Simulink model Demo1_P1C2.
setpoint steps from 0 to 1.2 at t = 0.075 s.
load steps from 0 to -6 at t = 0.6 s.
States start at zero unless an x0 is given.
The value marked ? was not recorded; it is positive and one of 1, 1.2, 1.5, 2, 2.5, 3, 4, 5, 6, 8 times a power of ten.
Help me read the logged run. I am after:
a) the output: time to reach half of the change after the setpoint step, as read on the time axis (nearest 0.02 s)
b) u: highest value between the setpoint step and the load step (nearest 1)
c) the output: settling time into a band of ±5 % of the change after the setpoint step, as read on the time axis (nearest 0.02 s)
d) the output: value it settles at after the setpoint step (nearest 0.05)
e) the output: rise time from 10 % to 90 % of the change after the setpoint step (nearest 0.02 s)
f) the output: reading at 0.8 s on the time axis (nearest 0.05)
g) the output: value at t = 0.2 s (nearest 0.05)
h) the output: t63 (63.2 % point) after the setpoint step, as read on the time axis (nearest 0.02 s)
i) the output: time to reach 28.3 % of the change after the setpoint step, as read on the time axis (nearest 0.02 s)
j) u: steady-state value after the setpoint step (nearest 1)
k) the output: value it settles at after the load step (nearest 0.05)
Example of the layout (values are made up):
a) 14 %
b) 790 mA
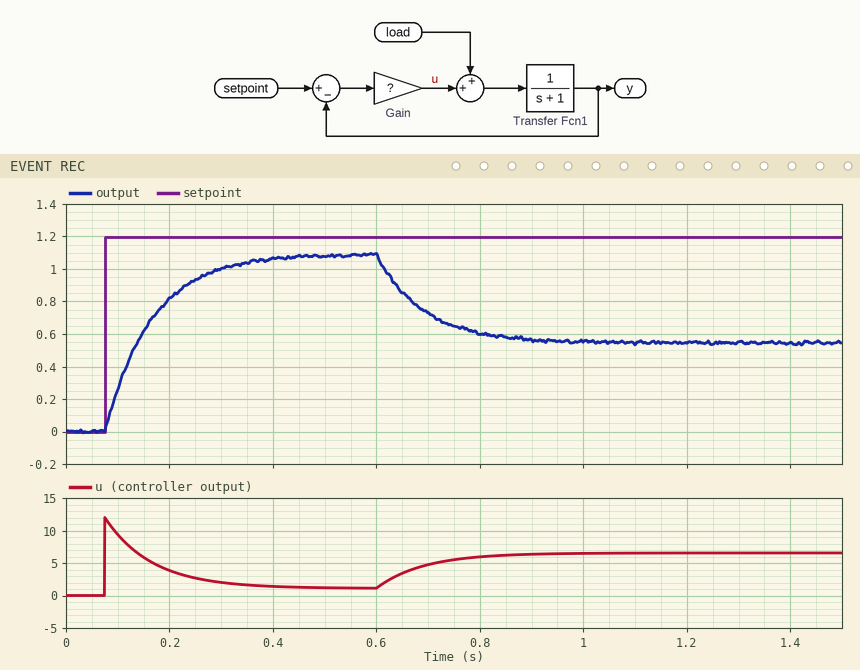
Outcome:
a) 0.14 s
b) 12
c) 0.34 s
d) 1.10
e) 0.20 s
f) 0.60
g) 0.80
h) 0.16 s
i) 0.10 s
j) 1
k) 0.55
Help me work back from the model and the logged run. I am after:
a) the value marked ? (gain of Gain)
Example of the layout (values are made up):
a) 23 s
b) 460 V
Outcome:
a) 10
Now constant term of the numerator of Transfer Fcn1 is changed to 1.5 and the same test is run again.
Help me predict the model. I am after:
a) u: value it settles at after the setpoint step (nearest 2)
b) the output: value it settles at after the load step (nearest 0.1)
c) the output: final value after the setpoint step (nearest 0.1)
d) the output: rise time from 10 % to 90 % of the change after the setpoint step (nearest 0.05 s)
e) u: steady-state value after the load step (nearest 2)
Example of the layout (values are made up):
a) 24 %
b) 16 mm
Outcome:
a) 0
b) 0.6
c) 1.1
d) 0.15 s
e) 6
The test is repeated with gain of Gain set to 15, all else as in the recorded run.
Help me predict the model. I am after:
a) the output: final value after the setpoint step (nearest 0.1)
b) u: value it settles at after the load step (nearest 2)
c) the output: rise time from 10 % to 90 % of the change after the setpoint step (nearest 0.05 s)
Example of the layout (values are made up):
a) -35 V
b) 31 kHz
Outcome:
a) 1.1
b) 6
c) 0.15 s
